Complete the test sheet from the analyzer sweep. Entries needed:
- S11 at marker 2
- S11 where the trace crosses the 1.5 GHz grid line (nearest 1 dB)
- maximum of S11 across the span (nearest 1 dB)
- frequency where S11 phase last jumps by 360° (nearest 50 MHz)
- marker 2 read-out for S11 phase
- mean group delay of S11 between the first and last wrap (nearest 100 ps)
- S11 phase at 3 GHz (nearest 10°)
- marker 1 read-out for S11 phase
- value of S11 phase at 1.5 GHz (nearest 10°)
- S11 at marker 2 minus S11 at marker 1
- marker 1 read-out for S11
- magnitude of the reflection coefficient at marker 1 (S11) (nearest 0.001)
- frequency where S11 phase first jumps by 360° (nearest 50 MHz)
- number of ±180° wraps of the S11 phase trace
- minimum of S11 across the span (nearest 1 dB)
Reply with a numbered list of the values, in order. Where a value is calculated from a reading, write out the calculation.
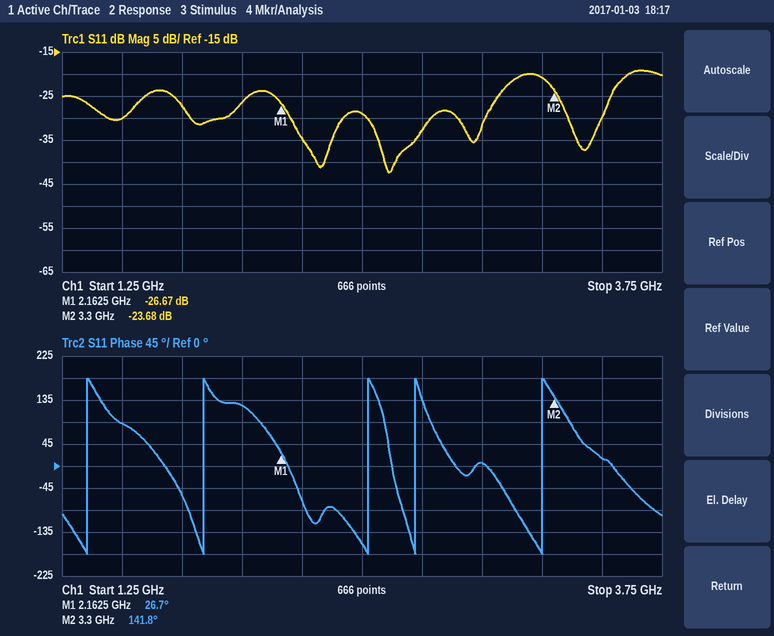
1. -23.68 dB
2. -30 dB
3. -19 dB
4. 3.25 GHz
5. 141.8°
6. 4 cycles / (3.25 GHz − 1.35 GHz) ≈ 2.1 ns
7. 10°
8. 26.7°
9. 90°
10. -23.68 − (-26.67) = 2.99 dB
11. -26.67 dB
12. 10^(-26.67/20) ≈ 0.046
13. 1.35 GHz
14. 5
15. -42 dB
